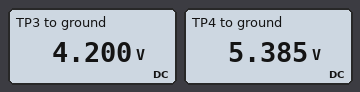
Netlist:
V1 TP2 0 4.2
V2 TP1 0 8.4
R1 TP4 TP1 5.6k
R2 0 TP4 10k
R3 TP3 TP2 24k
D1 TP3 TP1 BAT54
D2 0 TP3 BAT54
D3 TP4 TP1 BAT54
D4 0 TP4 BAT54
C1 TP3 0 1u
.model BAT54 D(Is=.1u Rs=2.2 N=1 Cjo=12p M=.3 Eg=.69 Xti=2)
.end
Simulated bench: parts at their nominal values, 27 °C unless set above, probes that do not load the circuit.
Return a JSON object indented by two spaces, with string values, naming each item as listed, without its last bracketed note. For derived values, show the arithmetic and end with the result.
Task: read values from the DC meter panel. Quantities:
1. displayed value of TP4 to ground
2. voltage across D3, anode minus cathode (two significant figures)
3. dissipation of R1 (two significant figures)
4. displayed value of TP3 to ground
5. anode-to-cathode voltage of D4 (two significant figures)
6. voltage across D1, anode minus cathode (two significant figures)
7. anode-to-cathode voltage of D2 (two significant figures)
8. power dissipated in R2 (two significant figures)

{
  "displayed value of TP4 to ground": "5.385 V",
  "voltage across D3, anode minus cathode": "5.385 V - 8.4 V = -3.0 V",
  "dissipation of R1": "(8.4 V - 5.385 V)^2 / 5.6 kΩ = 1.6 mW",
  "displayed value of TP3 to ground": "4.200 V",
  "anode-to-cathode voltage of D4": "0 V - 5.385 V = -5.4 V",
  "voltage across D1, anode minus cathode": "4.2 V - 8.4 V = -4.2 V",
  "anode-to-cathode voltage of D2": "0 V - 4.2 V = -4.2 V",
  "power dissipated in R2": "(5.385 V)^2 / 10 kΩ = 2.9 mW"
}
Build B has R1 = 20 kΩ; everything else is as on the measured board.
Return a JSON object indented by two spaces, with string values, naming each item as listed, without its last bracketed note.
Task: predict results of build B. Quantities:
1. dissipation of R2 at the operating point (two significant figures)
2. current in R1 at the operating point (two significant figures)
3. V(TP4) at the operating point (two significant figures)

{
  "dissipation of R2 at the operating point": "780 µW",
  "current in R1 at the operating point": "280 µA",
  "V(TP4) at the operating point": "2.8 V"
}
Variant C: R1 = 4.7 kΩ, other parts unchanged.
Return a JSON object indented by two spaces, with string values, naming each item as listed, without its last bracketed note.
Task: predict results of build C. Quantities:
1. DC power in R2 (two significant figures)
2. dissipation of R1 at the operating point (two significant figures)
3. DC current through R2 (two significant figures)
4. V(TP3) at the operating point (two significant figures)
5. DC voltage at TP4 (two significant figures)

{
  "DC power in R2": "3.3 mW",
  "dissipation of R1 at the operating point": "1.5 mW",
  "DC current through R2": "570 µA",
  "V(TP3) at the operating point": "4.2 V",
  "DC voltage at TP4": "5.7 V"
}
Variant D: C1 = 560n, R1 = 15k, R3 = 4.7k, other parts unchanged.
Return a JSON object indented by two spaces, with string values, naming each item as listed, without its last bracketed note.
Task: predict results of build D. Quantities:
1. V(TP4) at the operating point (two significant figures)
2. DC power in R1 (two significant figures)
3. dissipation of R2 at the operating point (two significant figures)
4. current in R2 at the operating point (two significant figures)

{
  "V(TP4) at the operating point": "3.4 V",
  "DC power in R1": "1.7 mW",
  "dissipation of R2 at the operating point": "1.1 mW",
  "current in R2 at the operating point": "340 µA"
}
